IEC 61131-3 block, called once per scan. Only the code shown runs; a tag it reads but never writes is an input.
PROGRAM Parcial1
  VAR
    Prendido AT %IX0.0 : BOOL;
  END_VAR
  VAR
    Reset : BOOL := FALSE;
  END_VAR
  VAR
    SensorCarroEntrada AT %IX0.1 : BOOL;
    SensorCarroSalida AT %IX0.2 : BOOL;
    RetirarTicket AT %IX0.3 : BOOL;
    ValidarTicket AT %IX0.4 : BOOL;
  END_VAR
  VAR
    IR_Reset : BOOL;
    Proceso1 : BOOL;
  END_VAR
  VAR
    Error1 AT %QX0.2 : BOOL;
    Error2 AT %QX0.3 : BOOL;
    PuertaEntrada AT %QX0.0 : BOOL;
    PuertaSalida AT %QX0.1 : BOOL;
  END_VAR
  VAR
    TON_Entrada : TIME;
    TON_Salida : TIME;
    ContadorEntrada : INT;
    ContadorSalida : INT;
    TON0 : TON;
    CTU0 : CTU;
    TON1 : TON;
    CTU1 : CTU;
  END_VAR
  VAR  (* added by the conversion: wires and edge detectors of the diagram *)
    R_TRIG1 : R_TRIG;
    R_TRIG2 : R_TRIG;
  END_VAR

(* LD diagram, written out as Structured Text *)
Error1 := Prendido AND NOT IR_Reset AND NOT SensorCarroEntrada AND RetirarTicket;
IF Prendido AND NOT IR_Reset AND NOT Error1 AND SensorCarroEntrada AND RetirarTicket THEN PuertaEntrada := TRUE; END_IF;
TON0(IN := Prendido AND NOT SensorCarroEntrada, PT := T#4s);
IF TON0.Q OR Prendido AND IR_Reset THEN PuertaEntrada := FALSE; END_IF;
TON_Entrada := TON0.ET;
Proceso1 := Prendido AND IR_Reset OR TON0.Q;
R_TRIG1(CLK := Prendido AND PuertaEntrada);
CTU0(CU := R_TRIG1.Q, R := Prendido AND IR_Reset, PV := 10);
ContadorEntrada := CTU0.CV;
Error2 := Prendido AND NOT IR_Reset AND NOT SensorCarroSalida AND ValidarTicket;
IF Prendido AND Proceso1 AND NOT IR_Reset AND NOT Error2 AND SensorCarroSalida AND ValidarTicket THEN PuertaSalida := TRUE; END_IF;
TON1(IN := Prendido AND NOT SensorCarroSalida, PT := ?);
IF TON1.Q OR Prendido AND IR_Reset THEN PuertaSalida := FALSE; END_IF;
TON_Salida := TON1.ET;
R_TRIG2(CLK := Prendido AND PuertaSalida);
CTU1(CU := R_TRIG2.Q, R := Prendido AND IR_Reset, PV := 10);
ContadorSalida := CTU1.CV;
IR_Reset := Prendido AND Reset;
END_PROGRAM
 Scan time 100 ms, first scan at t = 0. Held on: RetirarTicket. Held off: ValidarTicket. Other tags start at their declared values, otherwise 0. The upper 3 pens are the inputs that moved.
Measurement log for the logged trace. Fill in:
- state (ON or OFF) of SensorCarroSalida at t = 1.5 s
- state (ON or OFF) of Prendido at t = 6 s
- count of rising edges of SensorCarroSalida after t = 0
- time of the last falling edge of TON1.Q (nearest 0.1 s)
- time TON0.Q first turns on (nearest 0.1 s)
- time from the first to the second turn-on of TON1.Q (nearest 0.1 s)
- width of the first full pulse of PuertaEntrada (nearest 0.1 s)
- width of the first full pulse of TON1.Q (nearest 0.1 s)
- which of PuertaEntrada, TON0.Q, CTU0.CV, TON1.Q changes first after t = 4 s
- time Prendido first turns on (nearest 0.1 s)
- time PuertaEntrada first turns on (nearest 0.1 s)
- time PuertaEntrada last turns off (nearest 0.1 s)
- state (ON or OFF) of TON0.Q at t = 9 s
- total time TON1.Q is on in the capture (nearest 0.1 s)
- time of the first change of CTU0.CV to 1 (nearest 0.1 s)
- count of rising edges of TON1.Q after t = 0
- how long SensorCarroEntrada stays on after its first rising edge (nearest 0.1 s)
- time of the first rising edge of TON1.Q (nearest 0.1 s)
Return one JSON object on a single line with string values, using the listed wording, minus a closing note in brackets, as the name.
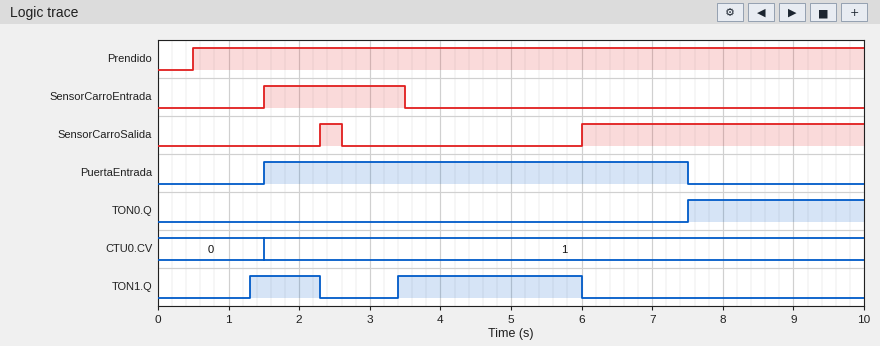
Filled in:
{"state (ON or OFF) of SensorCarroSalida at t = 1.5 s": "OFF", "state (ON or OFF) of Prendido at t = 6 s": "ON", "count of rising edges of SensorCarroSalida after t = 0": "2", "time of the last falling edge of TON1.Q": "6.0 s", "time TON0.Q first turns on": "7.5 s", "time from the first to the second turn-on of TON1.Q": "2.1 s", "width of the first full pulse of PuertaEntrada": "6.0 s", "width of the first full pulse of TON1.Q": "1.0 s", "which of PuertaEntrada, TON0.Q, CTU0.CV, TON1.Q changes first after t = 4 s": "TON1.Q", "time Prendido first turns on": "0.5 s", "time PuertaEntrada first turns on": "1.5 s", "time PuertaEntrada last turns off": "7.5 s", "state (ON or OFF) of TON0.Q at t = 9 s": "ON", "total time TON1.Q is on in the capture": "3.6 s", "time of the first change of CTU0.CV to 1": "1.5 s", "count of rising edges of TON1.Q after t = 0": "2", "how long SensorCarroEntrada stays on after its first rising edge": "2.0 s", "time of the first rising edge of TON1.Q": "1.3 s"}
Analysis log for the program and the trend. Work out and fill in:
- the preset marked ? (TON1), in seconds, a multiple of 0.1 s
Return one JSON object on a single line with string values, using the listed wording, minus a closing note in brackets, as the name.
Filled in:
{"the preset marked ? (TON1), in seconds, a multiple of 0.1 s": "0.8 s"}
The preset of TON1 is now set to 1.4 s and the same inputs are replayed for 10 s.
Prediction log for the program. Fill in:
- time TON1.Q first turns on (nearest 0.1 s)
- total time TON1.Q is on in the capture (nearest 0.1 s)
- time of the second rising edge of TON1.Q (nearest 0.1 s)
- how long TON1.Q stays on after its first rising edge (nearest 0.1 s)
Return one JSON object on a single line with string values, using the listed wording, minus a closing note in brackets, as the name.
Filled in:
{"time TON1.Q first turns on": "1.9 s", "total time TON1.Q is on in the capture": "2.4 s", "time of the second rising edge of TON1.Q": "4.0 s", "how long TON1.Q stays on after its first rising edge": "0.4 s"}
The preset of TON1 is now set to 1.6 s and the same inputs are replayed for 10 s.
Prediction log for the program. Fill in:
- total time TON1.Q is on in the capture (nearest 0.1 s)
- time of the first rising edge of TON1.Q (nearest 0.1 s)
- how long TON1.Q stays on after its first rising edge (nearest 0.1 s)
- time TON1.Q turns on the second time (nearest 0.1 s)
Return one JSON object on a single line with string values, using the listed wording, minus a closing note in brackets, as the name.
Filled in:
{"total time TON1.Q is on in the capture": "2.0 s", "time of the first rising edge of TON1.Q": "2.1 s", "how long TON1.Q stays on after its first rising edge": "0.2 s", "time TON1.Q turns on the second time": "4.2 s"}
